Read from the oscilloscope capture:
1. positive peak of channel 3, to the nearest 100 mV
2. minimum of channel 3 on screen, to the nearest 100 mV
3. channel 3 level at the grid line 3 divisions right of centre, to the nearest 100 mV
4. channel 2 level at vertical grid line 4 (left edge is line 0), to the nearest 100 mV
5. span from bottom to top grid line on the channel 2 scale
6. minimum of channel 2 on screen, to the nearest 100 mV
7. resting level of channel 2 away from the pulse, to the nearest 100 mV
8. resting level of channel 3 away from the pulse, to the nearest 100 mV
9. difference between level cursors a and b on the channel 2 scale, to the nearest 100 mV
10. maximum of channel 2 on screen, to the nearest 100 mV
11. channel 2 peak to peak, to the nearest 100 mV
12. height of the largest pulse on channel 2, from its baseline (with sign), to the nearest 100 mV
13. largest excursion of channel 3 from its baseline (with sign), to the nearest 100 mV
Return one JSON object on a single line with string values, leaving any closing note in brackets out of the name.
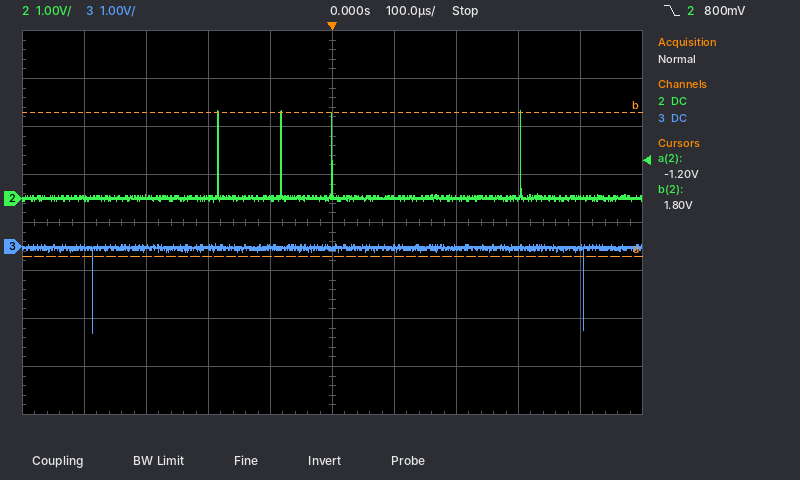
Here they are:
{"positive peak of channel 3, to the nearest 100 mV": "100 mV", "minimum of channel 3 on screen, to the nearest 100 mV": "-1.8 V", "channel 3 level at the grid line 3 divisions right of centre, to the nearest 100 mV": "0.0 V", "channel 2 level at vertical grid line 4 (left edge is line 0), to the nearest 100 mV": "0.0 V", "span from bottom to top grid line on the channel 2 scale": "8 V", "minimum of channel 2 on screen, to the nearest 100 mV": "-100 mV", "resting level of channel 2 away from the pulse, to the nearest 100 mV": "0.0 V", "resting level of channel 3 away from the pulse, to the nearest 100 mV": "0.0 V", "difference between level cursors a and b on the channel 2 scale, to the nearest 100 mV": "3.0 V", "maximum of channel 2 on screen, to the nearest 100 mV": "1.8 V", "channel 2 peak to peak, to the nearest 100 mV": "1.9 V", "height of the largest pulse on channel 2, from its baseline (with sign), to the nearest 100 mV": "+1.8 V", "largest excursion of channel 3 from its baseline (with sign), to the nearest 100 mV": "-1.8 V"}
